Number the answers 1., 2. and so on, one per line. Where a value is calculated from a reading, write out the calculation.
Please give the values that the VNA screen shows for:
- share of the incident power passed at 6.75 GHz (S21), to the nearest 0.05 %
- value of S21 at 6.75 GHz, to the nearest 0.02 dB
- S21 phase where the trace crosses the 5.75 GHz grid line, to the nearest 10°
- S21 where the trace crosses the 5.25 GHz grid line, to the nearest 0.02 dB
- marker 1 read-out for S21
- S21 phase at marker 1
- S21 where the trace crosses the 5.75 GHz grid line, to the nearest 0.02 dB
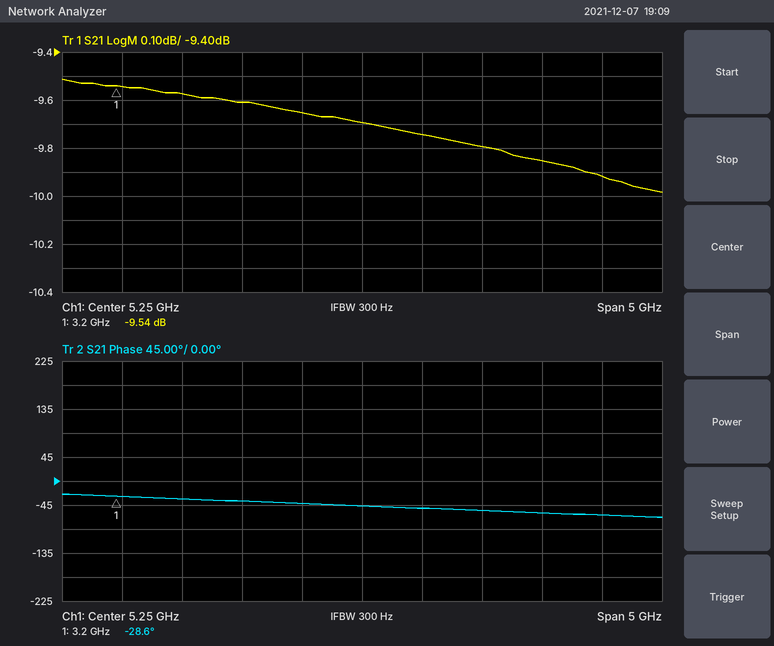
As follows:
1. 10^(-9.86/10) ≈ 10.3 %, so 10.35 % to the nearest 0.05 %
2. -9.86 dB
3. -50°
4. -9.70 dB
5. -9.54 dB
6. -28.6°
7. -9.74 dB
